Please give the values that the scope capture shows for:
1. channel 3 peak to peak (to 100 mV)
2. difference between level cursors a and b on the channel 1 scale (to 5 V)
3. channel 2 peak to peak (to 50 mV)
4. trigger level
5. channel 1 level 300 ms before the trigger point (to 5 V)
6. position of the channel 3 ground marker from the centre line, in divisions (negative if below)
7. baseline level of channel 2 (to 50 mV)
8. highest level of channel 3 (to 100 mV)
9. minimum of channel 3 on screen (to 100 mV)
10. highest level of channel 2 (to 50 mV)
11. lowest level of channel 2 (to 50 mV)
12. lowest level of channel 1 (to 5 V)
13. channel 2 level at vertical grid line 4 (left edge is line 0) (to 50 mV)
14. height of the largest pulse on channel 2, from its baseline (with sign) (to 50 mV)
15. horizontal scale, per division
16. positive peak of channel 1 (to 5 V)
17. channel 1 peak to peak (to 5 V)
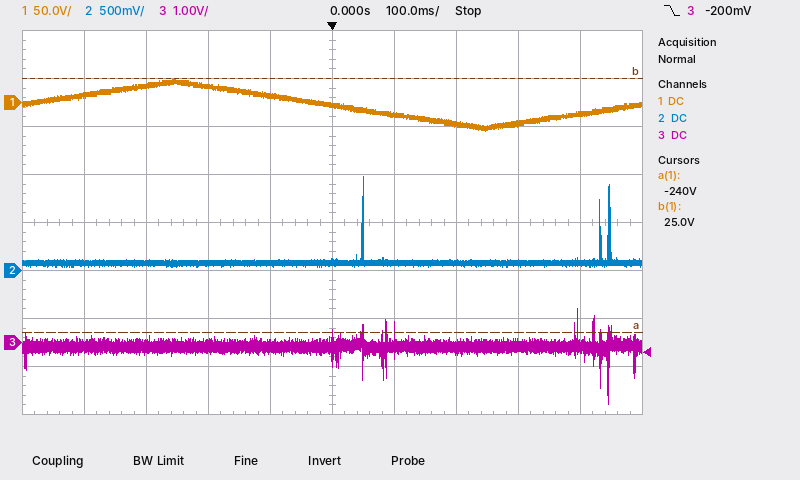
2.0 V
265 V
950 mV
-200 mV
20 V
-2.5 div
100 mV
700 mV
-1.3 V
1.00 V
50 mV
-30 V
100 mV
+900 mV
100 ms
25 V
55 V
